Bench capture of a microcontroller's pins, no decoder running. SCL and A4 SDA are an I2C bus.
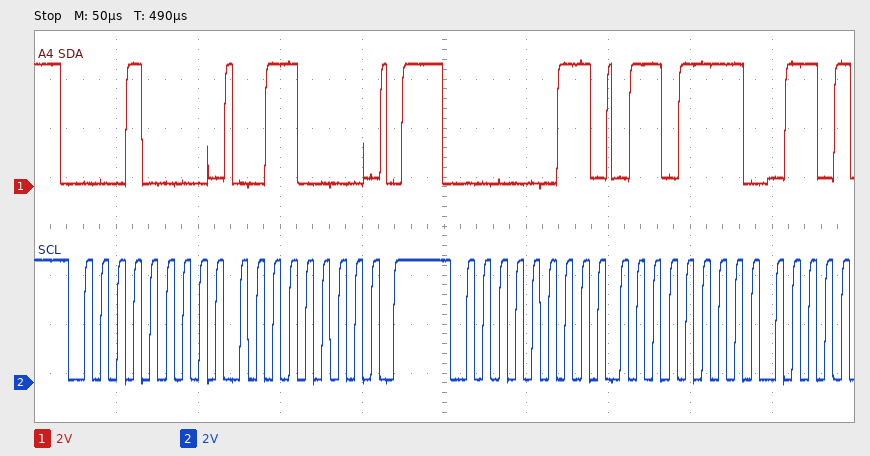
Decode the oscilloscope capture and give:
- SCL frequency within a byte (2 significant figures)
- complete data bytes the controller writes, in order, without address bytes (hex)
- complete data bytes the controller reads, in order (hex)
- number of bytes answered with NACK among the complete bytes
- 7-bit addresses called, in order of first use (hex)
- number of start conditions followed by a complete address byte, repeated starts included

100 kHz
30
6F
0
0x08 0x01
2
